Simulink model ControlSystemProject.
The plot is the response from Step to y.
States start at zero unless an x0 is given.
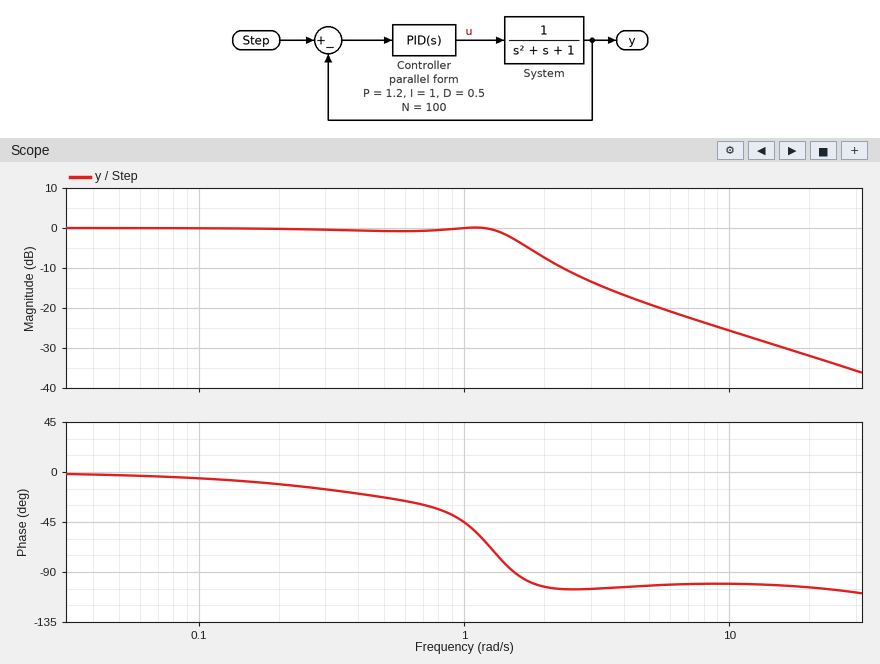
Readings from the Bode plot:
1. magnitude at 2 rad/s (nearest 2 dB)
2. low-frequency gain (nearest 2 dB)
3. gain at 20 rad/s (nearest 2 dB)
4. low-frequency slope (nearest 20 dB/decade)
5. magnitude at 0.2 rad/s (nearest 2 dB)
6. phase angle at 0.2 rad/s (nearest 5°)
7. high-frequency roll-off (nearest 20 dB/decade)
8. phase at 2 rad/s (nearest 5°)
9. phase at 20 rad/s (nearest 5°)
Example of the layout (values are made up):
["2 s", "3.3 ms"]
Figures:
["-8 dB", "0 dB", "-32 dB", "0 dB/decade", "0 dB", "-10°", "-20 dB/decade", "-105°", "-105°"]
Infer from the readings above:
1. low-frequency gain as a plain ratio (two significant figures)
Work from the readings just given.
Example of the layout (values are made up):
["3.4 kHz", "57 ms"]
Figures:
["1.0"]
